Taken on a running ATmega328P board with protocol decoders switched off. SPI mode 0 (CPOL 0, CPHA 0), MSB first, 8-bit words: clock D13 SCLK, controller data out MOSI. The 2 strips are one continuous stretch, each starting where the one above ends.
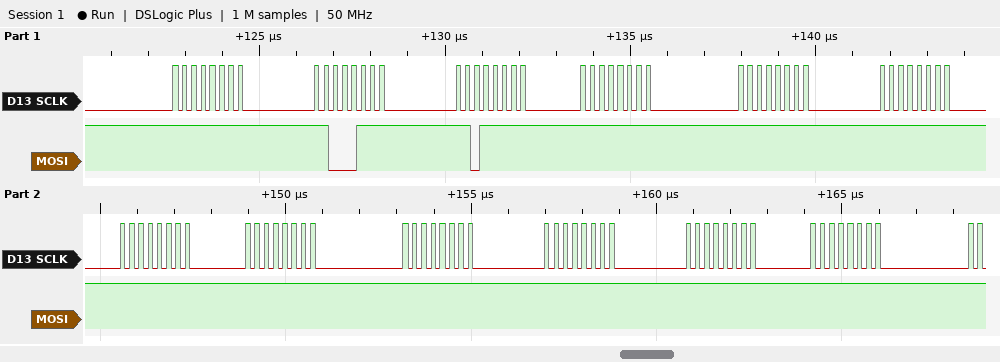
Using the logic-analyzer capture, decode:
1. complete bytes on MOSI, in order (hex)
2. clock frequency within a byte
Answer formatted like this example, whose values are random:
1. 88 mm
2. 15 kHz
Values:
1. FF C7 DF FF FF FF FF FF FF FF FF FF
2. 4 MHz
